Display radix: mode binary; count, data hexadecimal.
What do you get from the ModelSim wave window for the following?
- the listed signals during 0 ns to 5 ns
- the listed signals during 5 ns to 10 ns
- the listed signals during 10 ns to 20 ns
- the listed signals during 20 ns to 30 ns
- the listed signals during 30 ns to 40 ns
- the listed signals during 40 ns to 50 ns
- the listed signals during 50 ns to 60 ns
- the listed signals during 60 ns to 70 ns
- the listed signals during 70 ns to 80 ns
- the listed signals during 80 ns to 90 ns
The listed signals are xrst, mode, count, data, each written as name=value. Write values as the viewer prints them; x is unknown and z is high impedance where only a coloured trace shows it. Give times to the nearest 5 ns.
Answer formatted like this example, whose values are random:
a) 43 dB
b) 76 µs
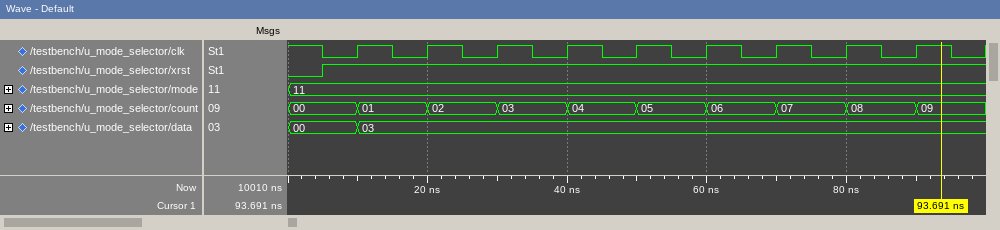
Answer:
a) xrst=0, mode=11, count=00, data=00
b) xrst=1, mode=11, count=00, data=00
c) xrst=1, mode=11, count=01, data=03
d) xrst=1, mode=11, count=02, data=03
e) xrst=1, mode=11, count=03, data=03
f) xrst=1, mode=11, count=04, data=03
g) xrst=1, mode=11, count=05, data=03
h) xrst=1, mode=11, count=06, data=03
i) xrst=1, mode=11, count=07, data=03
j) xrst=1, mode=11, count=08, data=03
